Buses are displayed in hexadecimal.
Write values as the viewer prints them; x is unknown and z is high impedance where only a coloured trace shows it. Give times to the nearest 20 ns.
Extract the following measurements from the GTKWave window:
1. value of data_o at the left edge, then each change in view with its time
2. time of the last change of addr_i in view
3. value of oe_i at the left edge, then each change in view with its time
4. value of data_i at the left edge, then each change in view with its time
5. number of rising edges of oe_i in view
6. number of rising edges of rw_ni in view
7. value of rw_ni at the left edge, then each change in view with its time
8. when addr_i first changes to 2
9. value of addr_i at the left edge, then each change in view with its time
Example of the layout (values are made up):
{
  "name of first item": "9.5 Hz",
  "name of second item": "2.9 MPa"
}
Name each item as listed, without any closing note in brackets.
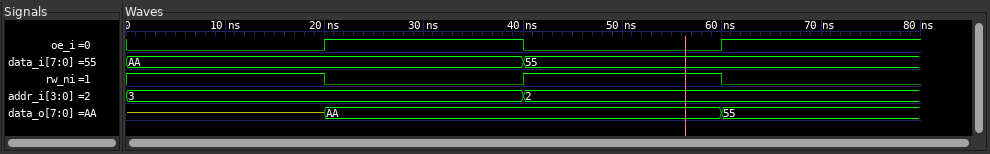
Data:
{
  "value of data_o at the left edge, then each change in view with its time": "z, AA at 20 ns, 55 at 60 ns",
  "time of the last change of addr_i in view": "40 ns",
  "value of oe_i at the left edge, then each change in view with its time": "0, 1 at 20 ns, 0 at 40 ns, 1 at 60 ns",
  "value of data_i at the left edge, then each change in view with its time": "AA, 55 at 40 ns",
  "number of rising edges of oe_i in view": "2",
  "number of rising edges of rw_ni in view": "1",
  "value of rw_ni at the left edge, then each change in view with its time": "1, 0 at 20 ns, 1 at 40 ns, 0 at 60 ns",
  "when addr_i first changes to 2": "40 ns",
  "value of addr_i at the left edge, then each change in view with its time": "3, 2 at 40 ns"
}
